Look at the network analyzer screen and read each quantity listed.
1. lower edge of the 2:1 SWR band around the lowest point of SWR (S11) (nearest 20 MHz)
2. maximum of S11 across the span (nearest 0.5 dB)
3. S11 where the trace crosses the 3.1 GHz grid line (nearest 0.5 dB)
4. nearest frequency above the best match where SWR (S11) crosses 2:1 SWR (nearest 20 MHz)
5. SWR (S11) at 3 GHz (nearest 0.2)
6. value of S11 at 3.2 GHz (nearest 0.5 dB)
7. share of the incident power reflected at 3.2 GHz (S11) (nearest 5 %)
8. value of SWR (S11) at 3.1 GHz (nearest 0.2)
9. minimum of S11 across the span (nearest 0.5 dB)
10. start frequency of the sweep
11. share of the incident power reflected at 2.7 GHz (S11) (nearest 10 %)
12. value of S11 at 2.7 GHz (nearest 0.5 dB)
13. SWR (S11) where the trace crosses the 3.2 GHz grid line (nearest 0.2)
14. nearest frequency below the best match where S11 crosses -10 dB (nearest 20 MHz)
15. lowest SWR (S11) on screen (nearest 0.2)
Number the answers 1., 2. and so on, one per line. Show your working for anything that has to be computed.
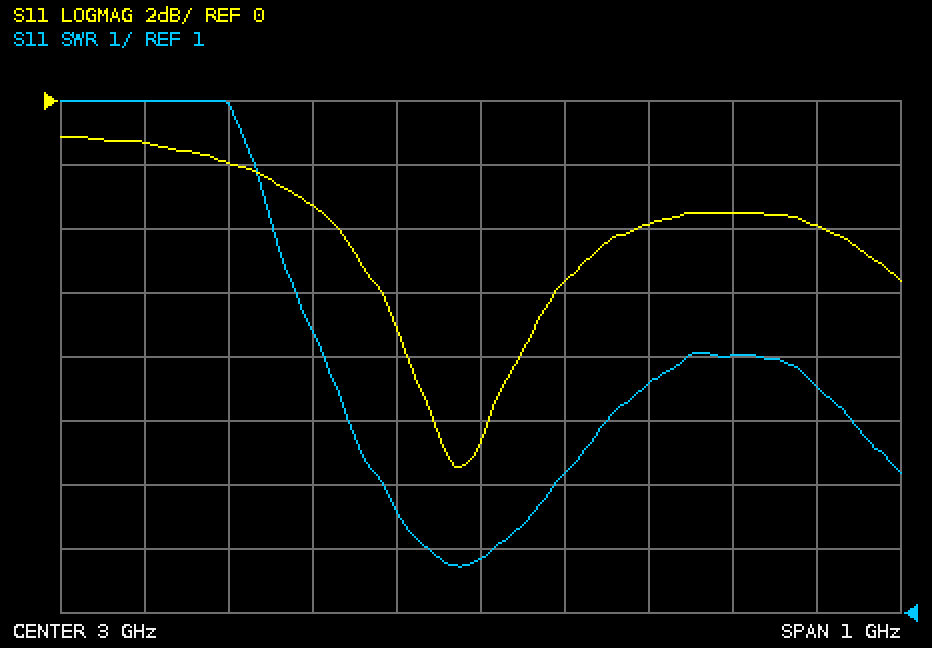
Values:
1. 2.94 GHz
2. -1.0 dB
3. -5.5 dB
4. 3.02 GHz
5. 1.8
6. -4.0 dB
7. 10^(-4/10) ≈ 40 %
8. 3.2
9. -11.5 dB
10. 2.5 GHz
11. 10^(-2/10) ≈ 63.1 %, so 60 % to the nearest 10 %
12. -2.0 dB
13. 4.6
14. 2.94 GHz
15. 1.8
